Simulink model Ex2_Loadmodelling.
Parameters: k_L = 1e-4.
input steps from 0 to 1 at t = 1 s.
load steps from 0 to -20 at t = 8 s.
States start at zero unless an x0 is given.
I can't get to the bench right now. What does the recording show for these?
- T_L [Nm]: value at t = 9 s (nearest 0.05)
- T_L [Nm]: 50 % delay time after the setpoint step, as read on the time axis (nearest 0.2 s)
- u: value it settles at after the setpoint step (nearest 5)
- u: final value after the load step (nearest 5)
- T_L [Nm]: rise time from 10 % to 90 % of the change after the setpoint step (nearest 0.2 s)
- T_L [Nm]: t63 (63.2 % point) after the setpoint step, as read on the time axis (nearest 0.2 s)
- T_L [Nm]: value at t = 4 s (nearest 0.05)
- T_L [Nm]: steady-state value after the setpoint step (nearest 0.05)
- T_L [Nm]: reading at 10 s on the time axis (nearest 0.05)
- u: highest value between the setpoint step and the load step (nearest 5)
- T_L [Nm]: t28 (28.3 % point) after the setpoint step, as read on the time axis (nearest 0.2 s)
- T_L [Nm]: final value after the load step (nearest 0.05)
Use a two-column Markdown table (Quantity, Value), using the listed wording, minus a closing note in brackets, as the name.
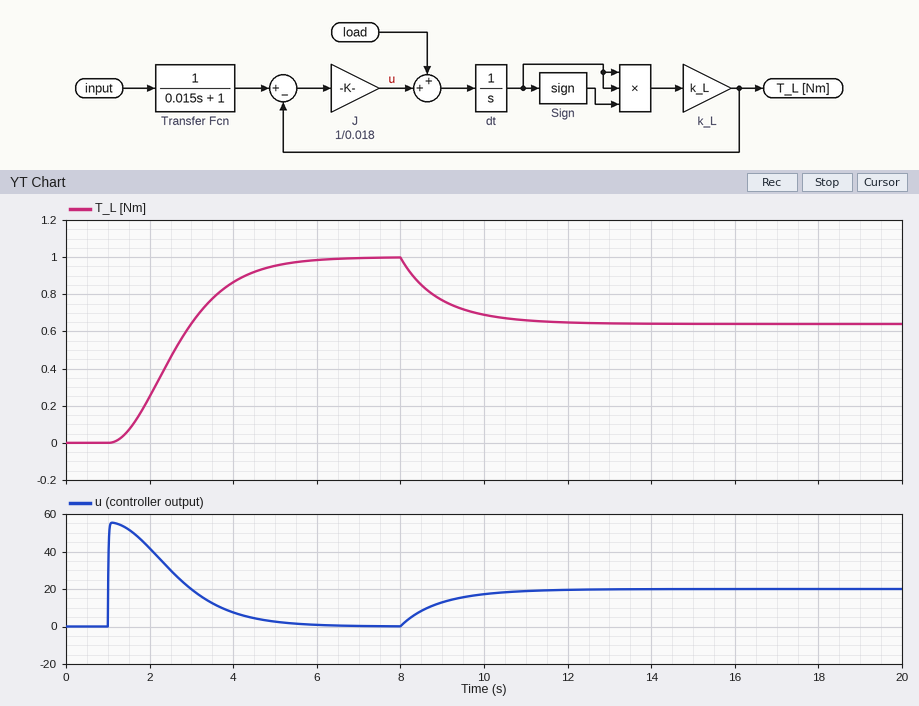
| Quantity | Value |
|---|---|
| T_L [Nm]: value at t = 9 s | 0.75 |
| T_L [Nm]: 50 % delay time after the setpoint step, as read on the time axis | 2.6 s |
| u: value it settles at after the setpoint step | 0 |
| u: final value after the load step | 20 |
| T_L [Nm]: rise time from 10 % to 90 % of the change after the setpoint step | 2.6 s |
| T_L [Nm]: t63 (63.2 % point) after the setpoint step, as read on the time axis | 3.0 s |
| T_L [Nm]: value at t = 4 s | 0.85 |
| T_L [Nm]: steady-state value after the setpoint step | 1.00 |
| T_L [Nm]: reading at 10 s on the time axis | 0.70 |
| u: highest value between the setpoint step and the load step | 55 |
| T_L [Nm]: t28 (28.3 % point) after the setpoint step, as read on the time axis | 2.0 s |
| T_L [Nm]: final value after the load step | 0.65 |
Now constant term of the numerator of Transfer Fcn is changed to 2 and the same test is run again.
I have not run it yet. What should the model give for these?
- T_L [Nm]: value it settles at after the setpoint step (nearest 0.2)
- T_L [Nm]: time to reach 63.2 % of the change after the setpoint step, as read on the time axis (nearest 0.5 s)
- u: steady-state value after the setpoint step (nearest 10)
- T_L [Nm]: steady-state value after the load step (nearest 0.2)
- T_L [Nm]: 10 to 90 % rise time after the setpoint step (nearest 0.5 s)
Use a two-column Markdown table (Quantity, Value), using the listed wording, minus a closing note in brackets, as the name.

| Quantity | Value |
|---|---|
| T_L [Nm]: value it settles at after the setpoint step | 2.0 |
| T_L [Nm]: time to reach 63.2 % of the change after the setpoint step, as read on the time axis | 2.5 s |
| u: steady-state value after the setpoint step | 0 |
| T_L [Nm]: steady-state value after the load step | 1.6 |
| T_L [Nm]: 10 to 90 % rise time after the setpoint step | 2.0 s |
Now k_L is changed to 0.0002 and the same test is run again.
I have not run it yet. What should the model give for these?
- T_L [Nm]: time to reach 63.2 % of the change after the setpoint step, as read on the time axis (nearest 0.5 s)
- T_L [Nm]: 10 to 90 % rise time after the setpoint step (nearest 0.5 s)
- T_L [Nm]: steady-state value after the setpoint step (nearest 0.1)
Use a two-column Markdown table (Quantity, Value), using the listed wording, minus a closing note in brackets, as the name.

| Quantity | Value |
|---|---|
| T_L [Nm]: time to reach 63.2 % of the change after the setpoint step, as read on the time axis | 2.5 s |
| T_L [Nm]: 10 to 90 % rise time after the setpoint step | 2.0 s |
| T_L [Nm]: steady-state value after the setpoint step | 1.0 |
